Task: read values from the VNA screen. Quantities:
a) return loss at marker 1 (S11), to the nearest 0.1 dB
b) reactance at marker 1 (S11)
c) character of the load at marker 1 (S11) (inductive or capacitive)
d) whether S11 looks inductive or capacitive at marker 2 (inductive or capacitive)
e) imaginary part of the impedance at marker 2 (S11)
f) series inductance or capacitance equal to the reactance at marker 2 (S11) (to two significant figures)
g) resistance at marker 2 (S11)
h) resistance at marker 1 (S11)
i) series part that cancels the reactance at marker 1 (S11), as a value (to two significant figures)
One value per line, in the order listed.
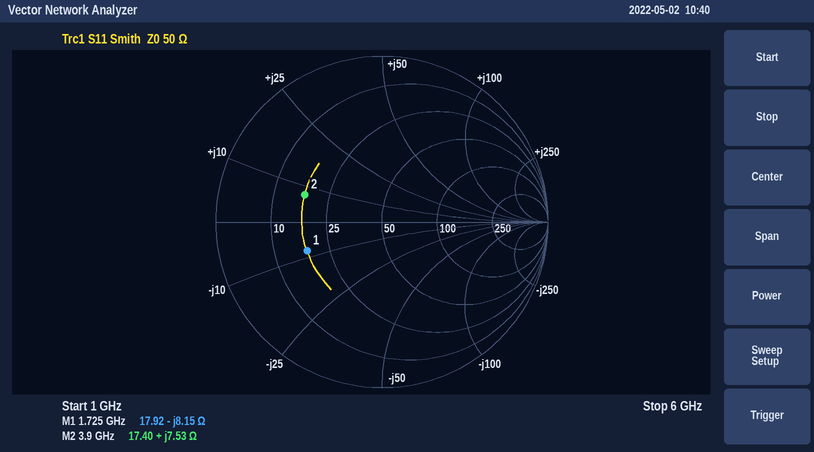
6.3 dB
-8.15 Ω
capacitive
inductive
+7.53 Ω
310 pH
17.40 Ω
17.92 Ω
750 pH
